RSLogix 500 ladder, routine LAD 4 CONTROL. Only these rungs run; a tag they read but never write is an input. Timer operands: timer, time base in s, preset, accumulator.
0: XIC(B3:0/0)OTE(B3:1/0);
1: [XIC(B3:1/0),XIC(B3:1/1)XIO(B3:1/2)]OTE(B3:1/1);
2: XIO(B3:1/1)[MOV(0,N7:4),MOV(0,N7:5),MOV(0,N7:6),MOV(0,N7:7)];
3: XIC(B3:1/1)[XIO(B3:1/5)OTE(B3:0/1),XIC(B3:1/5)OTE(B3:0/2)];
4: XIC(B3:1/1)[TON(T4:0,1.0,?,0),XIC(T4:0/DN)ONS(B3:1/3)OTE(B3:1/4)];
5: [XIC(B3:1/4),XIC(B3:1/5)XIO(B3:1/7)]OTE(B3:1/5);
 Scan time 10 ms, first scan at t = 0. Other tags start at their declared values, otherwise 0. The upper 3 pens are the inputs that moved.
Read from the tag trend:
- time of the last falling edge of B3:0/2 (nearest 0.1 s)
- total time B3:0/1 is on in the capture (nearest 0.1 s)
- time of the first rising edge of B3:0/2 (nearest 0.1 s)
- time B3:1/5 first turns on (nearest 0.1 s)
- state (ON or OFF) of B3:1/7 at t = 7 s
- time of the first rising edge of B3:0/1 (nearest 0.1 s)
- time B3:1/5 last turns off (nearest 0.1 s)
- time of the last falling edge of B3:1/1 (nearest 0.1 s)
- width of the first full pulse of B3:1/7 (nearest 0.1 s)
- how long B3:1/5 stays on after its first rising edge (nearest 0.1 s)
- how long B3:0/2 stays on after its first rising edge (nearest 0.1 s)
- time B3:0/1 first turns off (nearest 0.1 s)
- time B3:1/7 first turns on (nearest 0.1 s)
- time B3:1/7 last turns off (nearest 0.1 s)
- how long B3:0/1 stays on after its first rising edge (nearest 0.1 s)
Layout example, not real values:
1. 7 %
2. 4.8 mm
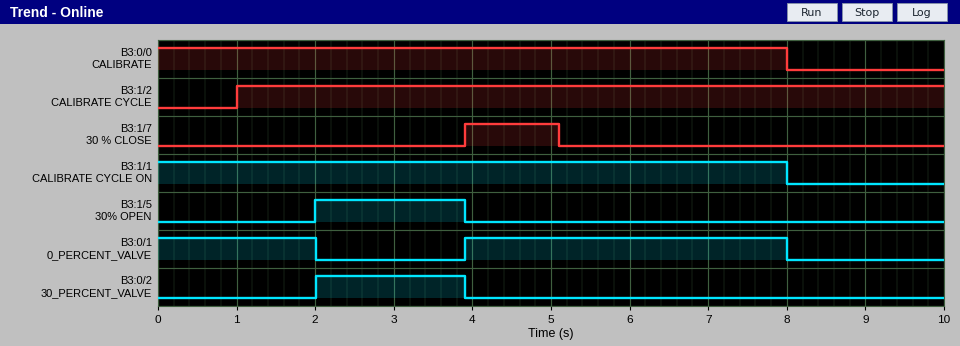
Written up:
1. 3.9 s
2. 6.1 s
3. 2.0 s
4. 2.0 s
5. OFF
6. 3.9 s
7. 3.9 s
8. 8.0 s
9. 1.2 s
10. 1.9 s
11. 1.9 s
12. 2.0 s
13. 3.9 s
14. 5.1 s
15. 4.1 s
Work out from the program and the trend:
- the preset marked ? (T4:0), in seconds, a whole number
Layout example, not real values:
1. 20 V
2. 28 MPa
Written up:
1. 2 s
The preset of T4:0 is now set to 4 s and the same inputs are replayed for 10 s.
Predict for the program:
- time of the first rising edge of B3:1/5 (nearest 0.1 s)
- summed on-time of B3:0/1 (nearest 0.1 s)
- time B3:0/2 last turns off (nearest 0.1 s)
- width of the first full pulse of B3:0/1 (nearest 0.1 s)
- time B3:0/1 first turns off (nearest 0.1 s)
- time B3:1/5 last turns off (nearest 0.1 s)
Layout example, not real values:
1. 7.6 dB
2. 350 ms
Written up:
1. 4.0 s
2. 8.0 s
3. 4.0 s
4. 4.0 s
5. 4.0 s
6. 4.0 s
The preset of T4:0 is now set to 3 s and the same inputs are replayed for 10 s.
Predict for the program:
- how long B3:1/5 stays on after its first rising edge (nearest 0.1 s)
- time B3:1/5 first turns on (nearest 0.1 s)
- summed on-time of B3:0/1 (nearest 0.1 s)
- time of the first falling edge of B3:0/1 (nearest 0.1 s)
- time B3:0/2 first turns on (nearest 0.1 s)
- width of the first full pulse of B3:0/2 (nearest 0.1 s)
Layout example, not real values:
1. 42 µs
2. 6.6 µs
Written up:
1. 0.9 s
2. 3.0 s
3. 7.1 s
4. 3.0 s
5. 3.0 s
6. 0.9 s
